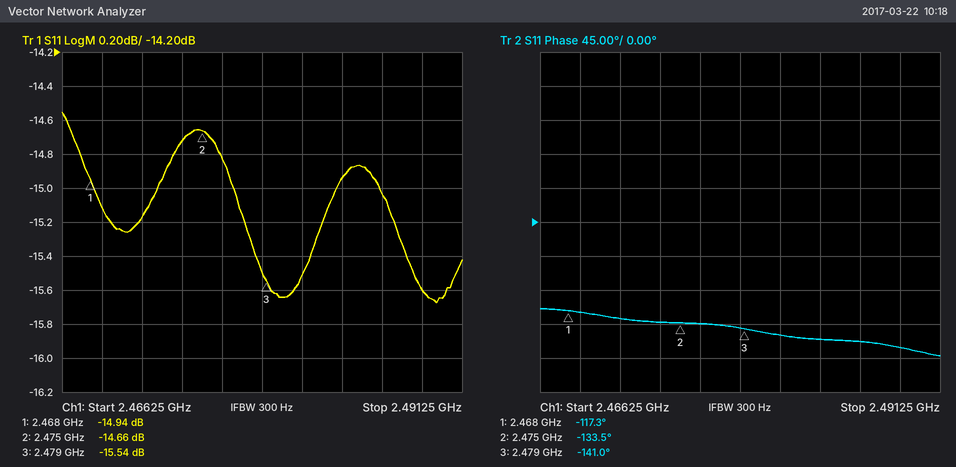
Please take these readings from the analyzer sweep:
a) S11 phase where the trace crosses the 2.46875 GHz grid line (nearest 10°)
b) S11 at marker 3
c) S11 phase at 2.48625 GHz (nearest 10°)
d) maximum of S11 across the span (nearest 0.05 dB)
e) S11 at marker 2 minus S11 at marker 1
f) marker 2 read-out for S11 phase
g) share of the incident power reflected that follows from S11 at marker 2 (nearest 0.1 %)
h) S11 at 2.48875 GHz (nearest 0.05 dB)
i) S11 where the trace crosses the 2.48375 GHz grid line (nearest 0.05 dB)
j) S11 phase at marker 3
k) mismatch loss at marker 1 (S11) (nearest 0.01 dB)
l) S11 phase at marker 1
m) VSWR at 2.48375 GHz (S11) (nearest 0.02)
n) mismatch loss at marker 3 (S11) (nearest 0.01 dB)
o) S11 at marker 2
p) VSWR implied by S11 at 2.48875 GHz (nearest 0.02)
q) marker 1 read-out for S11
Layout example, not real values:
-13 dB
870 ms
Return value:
-120°
-15.54 dB
-160°
-14.55 dB
0.28 dB
-133.5°
3.4 %
-15.60 dB
-14.95 dB
-141.0°
0.14 dB
-117.3°
1.44
0.12 dB
-14.66 dB
1.40
-14.94 dB
